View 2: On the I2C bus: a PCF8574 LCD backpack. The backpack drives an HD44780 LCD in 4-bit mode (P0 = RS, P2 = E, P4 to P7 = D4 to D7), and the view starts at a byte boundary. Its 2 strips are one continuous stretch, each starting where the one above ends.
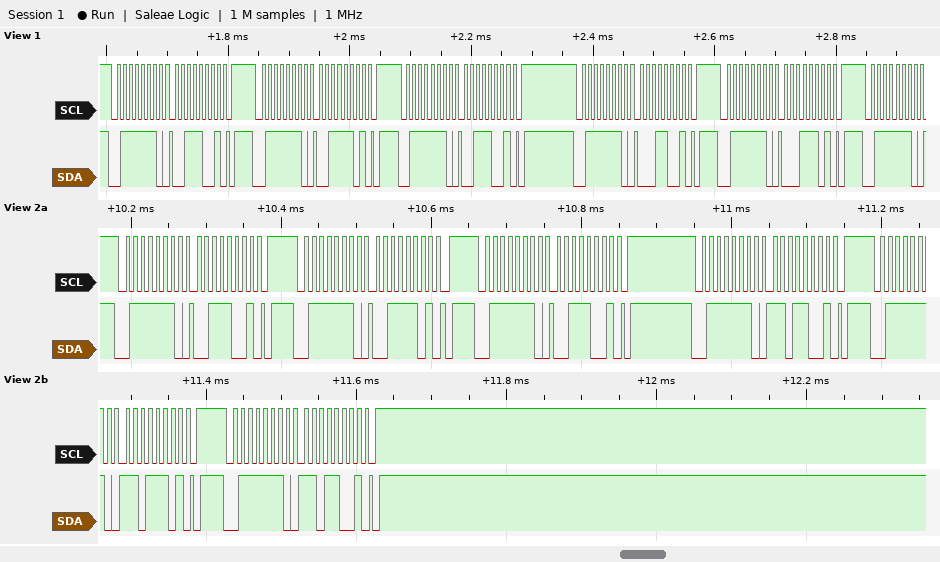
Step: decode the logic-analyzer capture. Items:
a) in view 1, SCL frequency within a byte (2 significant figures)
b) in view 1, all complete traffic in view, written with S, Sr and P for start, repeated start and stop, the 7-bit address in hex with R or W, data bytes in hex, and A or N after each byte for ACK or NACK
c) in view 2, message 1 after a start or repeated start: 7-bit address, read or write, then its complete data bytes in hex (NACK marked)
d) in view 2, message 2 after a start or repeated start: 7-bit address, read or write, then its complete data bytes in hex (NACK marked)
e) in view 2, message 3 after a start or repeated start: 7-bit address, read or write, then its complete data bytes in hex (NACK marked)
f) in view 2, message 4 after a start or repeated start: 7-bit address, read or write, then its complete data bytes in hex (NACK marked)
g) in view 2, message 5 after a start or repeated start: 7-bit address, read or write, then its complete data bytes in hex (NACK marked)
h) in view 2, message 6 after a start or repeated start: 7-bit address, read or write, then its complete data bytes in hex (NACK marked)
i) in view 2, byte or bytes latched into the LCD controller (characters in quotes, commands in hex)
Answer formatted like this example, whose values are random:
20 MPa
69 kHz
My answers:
100 kHz
S 3FW A 39 A P S 3FW A 3D A P S 3FW A 39 A P S 3FW A 19 A P S 3FW A 1D A P S 3FW A
0x3F write: 39
0x3F write: 3D
0x3F write: 39
0x3F write: D9
0x3F write: DD
0x3F write: D9
'='
